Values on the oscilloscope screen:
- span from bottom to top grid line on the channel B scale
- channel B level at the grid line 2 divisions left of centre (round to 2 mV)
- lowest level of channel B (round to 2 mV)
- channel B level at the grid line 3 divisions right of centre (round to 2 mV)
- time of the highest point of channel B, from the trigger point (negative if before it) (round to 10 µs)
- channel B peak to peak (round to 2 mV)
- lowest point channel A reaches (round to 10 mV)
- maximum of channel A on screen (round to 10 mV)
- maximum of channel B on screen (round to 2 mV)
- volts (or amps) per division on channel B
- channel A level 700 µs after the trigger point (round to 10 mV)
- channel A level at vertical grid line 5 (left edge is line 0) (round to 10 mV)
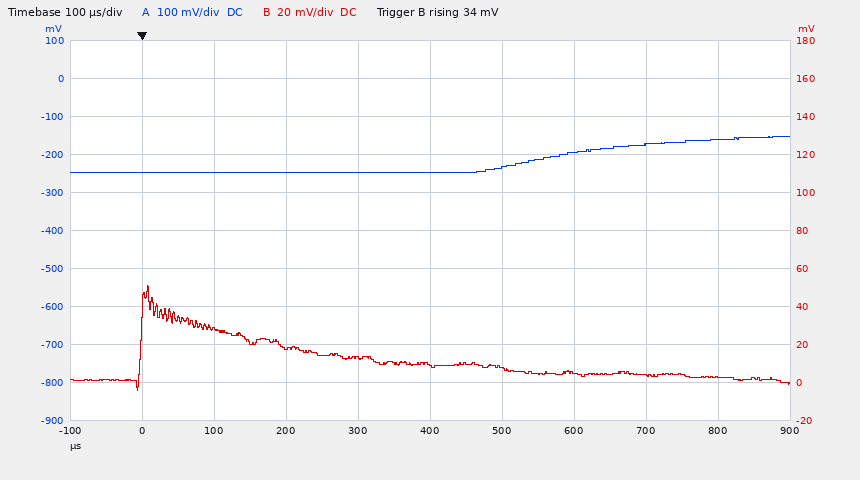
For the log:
200 mV
18 mV
-4 mV
4 mV
+10 µs
56 mV
-250 mV
-150 mV
52 mV
20 mV
-170 mV
-250 mV
